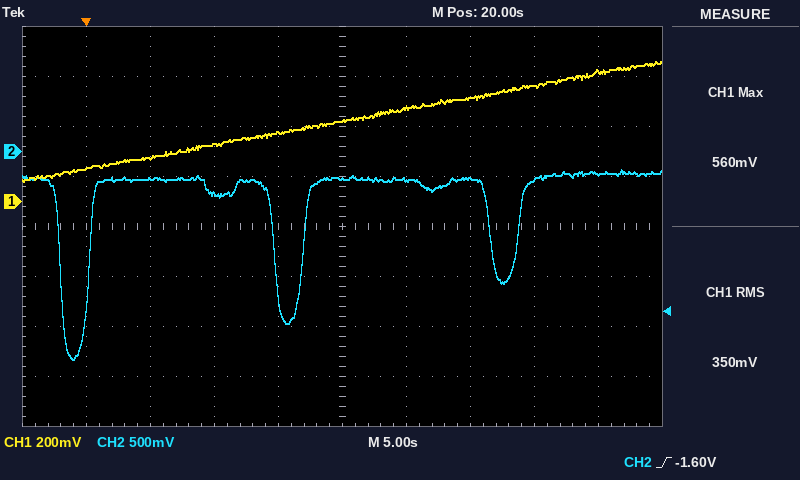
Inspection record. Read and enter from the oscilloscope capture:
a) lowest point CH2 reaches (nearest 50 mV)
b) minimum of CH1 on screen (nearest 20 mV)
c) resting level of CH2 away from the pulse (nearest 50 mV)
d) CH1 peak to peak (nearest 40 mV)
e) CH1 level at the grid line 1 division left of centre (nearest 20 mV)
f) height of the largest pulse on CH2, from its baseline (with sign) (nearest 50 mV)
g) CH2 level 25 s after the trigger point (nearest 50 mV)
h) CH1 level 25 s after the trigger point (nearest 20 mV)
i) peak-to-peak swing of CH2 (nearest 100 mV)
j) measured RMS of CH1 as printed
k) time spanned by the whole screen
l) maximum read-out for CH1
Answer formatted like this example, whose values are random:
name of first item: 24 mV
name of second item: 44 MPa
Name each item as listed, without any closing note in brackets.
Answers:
lowest point CH2 reaches: -2.10 V
minimum of CH1 on screen: 80 mV
resting level of CH2 away from the pulse: -300 mV
CH1 peak to peak: 480 mV
CH1 level at the grid line 1 division left of centre: 280 mV
height of the largest pulse on CH2, from its baseline (with sign): -1.80 V
CH2 level 25 s after the trigger point: -300 mV
CH1 level 25 s after the trigger point: 380 mV
peak-to-peak swing of CH2: 1.90 V
measured RMS of CH1 as printed: 350 mV
time spanned by the whole screen: 50 s
maximum read-out for CH1: 560 mV
